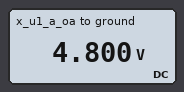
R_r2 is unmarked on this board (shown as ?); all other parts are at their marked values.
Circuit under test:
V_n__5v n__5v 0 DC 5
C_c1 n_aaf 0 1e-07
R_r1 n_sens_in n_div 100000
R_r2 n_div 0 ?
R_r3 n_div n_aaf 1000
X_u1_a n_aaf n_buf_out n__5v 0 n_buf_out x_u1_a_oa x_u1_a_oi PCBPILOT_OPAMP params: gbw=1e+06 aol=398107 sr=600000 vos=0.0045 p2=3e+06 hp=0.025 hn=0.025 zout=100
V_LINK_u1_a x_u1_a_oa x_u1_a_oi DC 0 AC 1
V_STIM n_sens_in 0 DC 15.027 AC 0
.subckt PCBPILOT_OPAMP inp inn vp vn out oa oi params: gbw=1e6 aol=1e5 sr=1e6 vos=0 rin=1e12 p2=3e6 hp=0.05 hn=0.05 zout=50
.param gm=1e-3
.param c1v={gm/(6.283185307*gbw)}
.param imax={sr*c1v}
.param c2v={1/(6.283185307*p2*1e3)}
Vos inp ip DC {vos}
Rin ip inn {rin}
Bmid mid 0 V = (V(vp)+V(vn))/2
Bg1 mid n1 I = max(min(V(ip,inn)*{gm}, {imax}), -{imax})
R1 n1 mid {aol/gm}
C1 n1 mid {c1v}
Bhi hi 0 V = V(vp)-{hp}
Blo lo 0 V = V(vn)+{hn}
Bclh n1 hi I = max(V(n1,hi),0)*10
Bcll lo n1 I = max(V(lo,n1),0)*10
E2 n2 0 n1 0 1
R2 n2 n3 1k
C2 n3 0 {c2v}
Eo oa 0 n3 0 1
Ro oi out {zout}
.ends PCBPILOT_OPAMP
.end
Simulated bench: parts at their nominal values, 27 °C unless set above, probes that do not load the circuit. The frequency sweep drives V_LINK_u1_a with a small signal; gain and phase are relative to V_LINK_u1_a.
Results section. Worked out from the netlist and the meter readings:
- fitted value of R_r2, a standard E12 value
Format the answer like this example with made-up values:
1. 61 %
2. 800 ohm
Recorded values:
1. 47 kΩ
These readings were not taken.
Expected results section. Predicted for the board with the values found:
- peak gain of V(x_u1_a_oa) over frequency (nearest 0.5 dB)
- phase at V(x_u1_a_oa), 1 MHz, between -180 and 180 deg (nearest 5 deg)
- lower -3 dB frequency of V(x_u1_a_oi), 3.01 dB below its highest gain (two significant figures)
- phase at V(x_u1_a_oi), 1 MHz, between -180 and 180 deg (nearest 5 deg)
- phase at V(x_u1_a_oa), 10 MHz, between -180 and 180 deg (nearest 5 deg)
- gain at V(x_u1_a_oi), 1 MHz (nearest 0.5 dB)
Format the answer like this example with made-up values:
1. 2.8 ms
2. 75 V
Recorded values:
1. 0 dB
2. -55 deg
3. 950 kHz
4. -130 deg
5. -165 deg
6. -1.0 dB
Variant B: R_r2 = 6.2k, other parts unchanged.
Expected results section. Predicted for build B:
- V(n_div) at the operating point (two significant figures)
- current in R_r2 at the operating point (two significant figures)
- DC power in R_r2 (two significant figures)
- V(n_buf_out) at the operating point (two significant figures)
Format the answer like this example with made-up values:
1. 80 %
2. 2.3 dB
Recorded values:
1. 880 mV
2. 140 µA
3. 120 µW
4. 870 mV
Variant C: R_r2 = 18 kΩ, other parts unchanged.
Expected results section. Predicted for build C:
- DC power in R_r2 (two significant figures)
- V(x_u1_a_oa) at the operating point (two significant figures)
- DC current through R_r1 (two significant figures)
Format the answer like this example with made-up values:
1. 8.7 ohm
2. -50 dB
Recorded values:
1. 290 µW
2. 2.3 V
3. 130 µA
